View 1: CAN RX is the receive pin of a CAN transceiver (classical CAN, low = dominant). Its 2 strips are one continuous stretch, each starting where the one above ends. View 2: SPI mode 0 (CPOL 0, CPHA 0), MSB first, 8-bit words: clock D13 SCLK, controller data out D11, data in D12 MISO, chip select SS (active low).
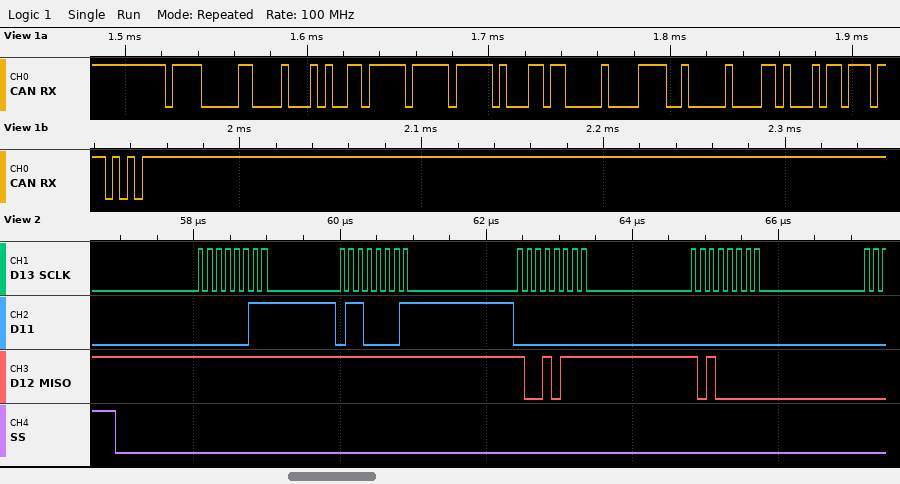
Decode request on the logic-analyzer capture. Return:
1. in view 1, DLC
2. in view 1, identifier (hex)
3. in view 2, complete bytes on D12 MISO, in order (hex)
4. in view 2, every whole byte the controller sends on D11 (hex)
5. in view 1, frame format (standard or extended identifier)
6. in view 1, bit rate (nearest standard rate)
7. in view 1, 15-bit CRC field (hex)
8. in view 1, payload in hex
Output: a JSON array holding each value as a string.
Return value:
["8", "0x782", "FF FF 97 A0", "03 61 00 00", "standard", "250 kbit/s", "0x5BBA", "A6 FF FF 1B 00 79 00 68"]
